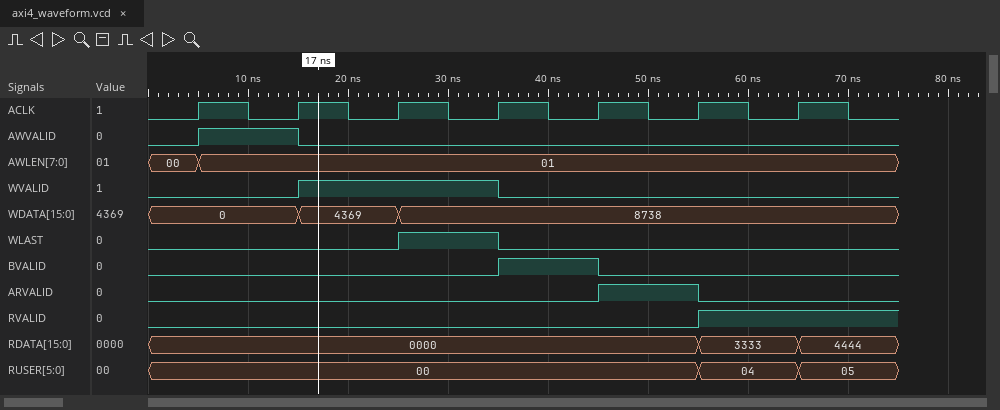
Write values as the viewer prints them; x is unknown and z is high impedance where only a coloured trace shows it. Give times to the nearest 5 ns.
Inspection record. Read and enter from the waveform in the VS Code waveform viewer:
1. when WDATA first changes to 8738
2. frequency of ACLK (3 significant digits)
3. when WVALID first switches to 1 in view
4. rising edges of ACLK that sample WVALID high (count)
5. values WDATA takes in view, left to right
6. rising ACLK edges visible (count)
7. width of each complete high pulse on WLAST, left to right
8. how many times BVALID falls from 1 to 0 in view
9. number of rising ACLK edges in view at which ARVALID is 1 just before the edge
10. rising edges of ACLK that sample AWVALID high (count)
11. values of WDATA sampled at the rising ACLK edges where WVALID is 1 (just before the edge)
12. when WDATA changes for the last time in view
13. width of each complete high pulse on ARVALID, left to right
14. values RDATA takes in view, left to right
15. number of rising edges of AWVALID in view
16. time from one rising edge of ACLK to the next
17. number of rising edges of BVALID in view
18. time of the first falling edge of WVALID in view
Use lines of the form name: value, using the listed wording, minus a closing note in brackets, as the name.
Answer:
when WDATA first changes to 8738: 25 ns
frequency of ACLK: 100 MHz
when WVALID first switches to 1 in view: 15 ns
rising edges of ACLK that sample WVALID high: 2
values WDATA takes in view, left to right: 0, 4369, 8738
rising ACLK edges visible: 7
width of each complete high pulse on WLAST, left to right: 10 ns
how many times BVALID falls from 1 to 0 in view: 1
number of rising ACLK edges in view at which ARVALID is 1 just before the edge: 1
rising edges of ACLK that sample AWVALID high: 1
values of WDATA sampled at the rising ACLK edges where WVALID is 1: 4369, 8738
when WDATA changes for the last time in view: 25 ns
width of each complete high pulse on ARVALID, left to right: 10 ns
values RDATA takes in view, left to right: 0000, 3333, 4444
number of rising edges of AWVALID in view: 1
time from one rising edge of ACLK to the next: 10 ns
number of rising edges of BVALID in view: 1
time of the first falling edge of WVALID in view: 35 ns
